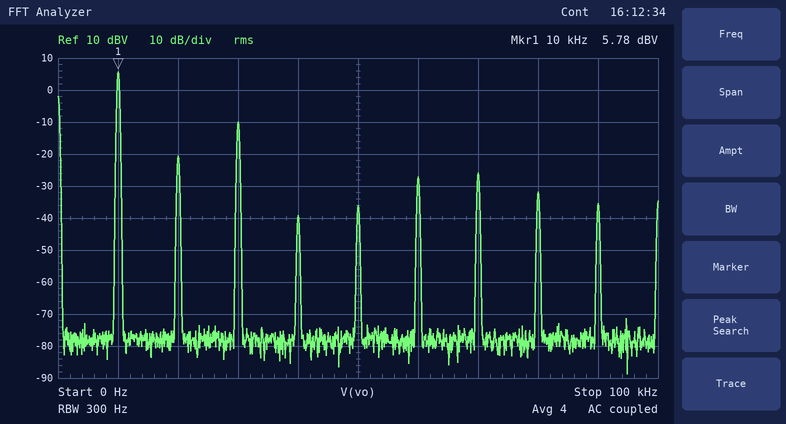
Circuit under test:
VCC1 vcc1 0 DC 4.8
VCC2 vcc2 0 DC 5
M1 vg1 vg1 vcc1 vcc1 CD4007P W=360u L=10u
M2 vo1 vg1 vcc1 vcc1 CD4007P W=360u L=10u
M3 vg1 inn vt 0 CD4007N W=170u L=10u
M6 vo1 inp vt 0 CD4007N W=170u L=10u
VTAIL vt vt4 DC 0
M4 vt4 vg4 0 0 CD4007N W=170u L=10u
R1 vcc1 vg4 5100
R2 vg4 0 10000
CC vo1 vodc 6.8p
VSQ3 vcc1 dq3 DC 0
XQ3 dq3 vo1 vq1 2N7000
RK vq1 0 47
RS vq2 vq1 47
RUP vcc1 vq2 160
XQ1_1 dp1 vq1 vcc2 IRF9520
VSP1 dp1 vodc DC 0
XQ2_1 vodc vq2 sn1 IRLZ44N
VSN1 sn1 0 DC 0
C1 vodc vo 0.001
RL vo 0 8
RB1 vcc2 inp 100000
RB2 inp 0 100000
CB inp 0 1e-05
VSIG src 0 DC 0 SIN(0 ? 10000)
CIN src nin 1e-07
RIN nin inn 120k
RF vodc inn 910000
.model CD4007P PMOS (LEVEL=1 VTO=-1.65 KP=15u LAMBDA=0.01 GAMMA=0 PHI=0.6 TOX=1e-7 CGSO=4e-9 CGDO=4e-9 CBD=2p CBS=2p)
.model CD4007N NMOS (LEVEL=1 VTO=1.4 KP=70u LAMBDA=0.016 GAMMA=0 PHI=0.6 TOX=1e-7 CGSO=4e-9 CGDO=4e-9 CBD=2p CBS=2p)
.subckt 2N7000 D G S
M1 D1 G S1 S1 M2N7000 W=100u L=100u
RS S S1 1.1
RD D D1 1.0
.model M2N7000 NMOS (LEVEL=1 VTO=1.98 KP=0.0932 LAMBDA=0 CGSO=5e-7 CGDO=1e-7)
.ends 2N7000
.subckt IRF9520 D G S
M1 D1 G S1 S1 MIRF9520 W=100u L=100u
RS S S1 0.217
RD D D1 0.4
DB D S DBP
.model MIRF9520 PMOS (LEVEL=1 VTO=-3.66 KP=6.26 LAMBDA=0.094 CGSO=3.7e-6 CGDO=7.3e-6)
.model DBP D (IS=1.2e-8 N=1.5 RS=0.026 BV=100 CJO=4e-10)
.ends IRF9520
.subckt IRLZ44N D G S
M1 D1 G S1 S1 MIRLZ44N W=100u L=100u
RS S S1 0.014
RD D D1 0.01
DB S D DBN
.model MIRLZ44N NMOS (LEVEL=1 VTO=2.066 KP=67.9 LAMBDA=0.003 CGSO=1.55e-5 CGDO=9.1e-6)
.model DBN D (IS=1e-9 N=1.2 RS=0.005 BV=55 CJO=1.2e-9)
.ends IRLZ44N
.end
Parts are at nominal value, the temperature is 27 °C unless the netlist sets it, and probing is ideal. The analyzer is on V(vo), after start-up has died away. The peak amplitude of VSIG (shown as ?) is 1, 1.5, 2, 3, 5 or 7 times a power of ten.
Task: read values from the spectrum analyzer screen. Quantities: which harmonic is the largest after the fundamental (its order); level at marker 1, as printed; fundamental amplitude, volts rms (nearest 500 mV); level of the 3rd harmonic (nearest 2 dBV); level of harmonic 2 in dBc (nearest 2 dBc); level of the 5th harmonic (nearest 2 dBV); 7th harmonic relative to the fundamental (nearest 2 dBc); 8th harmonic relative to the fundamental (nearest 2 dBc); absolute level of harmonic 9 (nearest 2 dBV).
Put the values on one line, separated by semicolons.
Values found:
3; 5.78 dBV; 2.0 V; -10 dBV; -26 dBc; -36 dBV; -32 dBc; -38 dBc; -36 dBV
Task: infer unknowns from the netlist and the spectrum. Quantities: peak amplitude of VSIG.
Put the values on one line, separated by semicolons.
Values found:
500 mV
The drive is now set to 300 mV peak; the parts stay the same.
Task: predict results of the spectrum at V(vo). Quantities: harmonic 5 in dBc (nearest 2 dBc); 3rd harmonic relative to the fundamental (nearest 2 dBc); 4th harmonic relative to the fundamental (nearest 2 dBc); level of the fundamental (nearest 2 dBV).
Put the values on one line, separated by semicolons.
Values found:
-50 dBc; -56 dBc; -50 dBc; 4 dBV
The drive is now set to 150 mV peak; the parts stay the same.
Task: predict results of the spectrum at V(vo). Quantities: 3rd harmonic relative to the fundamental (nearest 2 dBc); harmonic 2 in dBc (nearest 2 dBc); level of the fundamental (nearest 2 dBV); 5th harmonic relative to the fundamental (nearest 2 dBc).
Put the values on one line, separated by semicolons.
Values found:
-52 dBc; -40 dBc; -2 dBV; -58 dBc
